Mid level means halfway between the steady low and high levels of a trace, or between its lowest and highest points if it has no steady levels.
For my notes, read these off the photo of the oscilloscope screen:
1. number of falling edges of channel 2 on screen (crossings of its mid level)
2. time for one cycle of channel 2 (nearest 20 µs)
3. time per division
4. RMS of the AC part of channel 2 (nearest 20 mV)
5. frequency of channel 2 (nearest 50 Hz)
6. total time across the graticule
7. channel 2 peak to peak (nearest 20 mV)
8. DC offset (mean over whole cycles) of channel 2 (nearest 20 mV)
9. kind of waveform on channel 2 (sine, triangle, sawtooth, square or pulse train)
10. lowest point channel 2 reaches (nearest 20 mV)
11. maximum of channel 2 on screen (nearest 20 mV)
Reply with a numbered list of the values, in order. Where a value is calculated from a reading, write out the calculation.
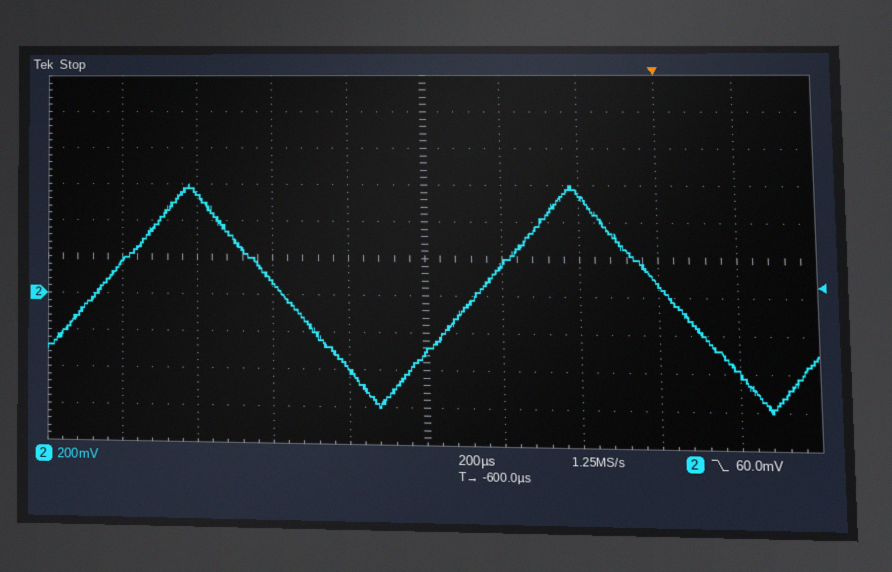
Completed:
1. 2
2. 1.00 ms
3. 200 µs
4. 1.20 V / (2√3) ≈ 346 mV, so 340 mV to the nearest 20 mV
5. 1 / 1.00 ms ≈ 1.00 kHz
6. 2 ms
7. 600 mV − (-600 mV) = 1.20 V
8. (600 mV + (-600 mV)) / 2 ≈ 0 mV
9. triangle
10. -600 mV
11. 600 mV
